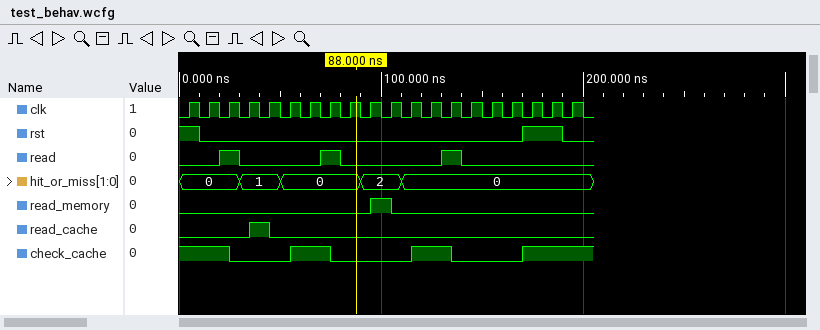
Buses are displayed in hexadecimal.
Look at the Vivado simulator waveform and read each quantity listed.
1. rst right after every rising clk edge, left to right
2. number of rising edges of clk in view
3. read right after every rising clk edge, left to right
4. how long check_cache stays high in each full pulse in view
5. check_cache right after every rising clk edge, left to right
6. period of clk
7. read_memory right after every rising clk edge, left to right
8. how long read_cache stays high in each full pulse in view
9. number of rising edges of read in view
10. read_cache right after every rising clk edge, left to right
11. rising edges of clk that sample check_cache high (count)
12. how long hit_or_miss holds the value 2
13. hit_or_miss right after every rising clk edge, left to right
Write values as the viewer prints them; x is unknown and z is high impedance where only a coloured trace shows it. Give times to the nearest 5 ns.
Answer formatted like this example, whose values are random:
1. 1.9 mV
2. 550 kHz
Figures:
1. 1 0 0 0 0 0 0 0 0 0 0 0 0 0 0 0 0 1 1 0
2. 20
3. 0 0 1 0 0 0 0 1 0 0 0 0 0 1 0 0 0 0 0 0
4. 20 ns, 20 ns
5. 1 1 0 0 0 1 1 0 0 0 0 1 1 0 0 0 0 1 1 1
6. 10 ns
7. 0 0 0 0 0 0 0 0 0 1 0 0 0 0 0 0 0 0 0 0
8. 10 ns
9. 3
10. 0 0 0 1 0 0 0 0 0 0 0 0 0 0 0 0 0 0 0 0
11. 10
12. 20 ns
13. 0, 0, 0, 1, 1, 0, 0, 0, 0, 2, 2, 0, 0, 0, 0, 0, 0, 0, 0, 0
